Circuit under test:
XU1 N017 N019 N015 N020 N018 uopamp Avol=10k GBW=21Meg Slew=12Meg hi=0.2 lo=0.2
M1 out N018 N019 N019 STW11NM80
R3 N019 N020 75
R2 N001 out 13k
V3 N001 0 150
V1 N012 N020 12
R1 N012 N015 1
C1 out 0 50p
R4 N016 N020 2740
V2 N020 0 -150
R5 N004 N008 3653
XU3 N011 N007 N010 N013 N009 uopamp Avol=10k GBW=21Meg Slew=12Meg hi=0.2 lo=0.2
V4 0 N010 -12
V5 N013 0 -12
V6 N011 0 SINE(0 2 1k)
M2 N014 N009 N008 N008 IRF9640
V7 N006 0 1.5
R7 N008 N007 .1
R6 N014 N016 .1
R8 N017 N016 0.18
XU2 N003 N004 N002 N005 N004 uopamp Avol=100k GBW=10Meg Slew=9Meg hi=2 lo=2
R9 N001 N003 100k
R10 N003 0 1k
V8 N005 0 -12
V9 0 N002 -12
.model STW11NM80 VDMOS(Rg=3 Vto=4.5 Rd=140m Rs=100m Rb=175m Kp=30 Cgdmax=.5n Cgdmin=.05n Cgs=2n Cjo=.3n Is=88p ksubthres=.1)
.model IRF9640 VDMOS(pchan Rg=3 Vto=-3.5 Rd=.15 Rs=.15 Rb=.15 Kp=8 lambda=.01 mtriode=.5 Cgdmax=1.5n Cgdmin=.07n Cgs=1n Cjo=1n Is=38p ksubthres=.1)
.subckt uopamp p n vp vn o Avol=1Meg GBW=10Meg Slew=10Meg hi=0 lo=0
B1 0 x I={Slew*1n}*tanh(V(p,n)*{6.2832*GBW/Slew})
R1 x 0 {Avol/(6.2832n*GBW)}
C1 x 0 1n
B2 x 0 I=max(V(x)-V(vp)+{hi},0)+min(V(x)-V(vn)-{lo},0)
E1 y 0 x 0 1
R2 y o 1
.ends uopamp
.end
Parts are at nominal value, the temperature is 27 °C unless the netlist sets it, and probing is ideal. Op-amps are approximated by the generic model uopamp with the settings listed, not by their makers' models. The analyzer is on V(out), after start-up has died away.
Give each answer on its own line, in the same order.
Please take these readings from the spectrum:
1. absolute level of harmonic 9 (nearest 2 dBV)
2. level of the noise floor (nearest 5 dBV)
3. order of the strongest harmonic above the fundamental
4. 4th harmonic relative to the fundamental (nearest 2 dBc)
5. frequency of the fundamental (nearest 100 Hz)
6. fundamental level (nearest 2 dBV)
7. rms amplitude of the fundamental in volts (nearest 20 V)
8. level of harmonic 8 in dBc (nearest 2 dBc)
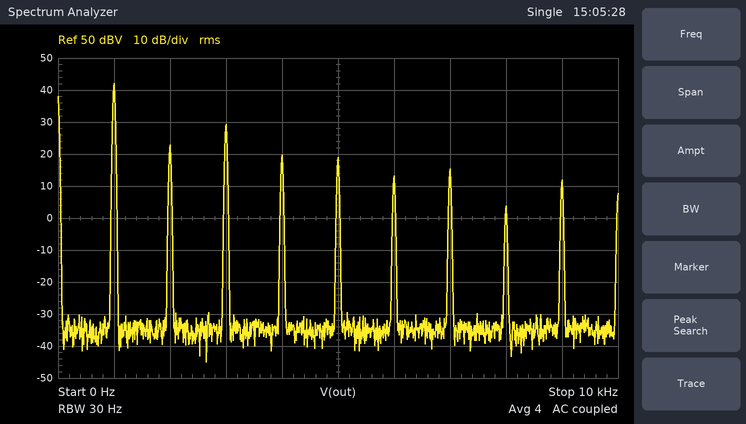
12 dBV
-35 dBV
3
-22 dBc
1.0 kHz
42 dBV
120 V
-38 dBc
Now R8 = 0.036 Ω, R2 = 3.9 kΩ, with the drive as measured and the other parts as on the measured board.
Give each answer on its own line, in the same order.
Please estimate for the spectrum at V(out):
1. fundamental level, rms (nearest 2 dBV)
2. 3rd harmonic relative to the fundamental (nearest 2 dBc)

34 dBV
-20 dBc
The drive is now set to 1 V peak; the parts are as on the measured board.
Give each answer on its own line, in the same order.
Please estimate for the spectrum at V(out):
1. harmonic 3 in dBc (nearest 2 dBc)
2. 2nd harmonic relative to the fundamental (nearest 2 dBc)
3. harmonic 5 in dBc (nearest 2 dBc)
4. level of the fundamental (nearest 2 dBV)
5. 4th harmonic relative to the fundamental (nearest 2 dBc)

-28 dBc
-26 dBc
-34 dBc
38 dBV
-30 dBc
